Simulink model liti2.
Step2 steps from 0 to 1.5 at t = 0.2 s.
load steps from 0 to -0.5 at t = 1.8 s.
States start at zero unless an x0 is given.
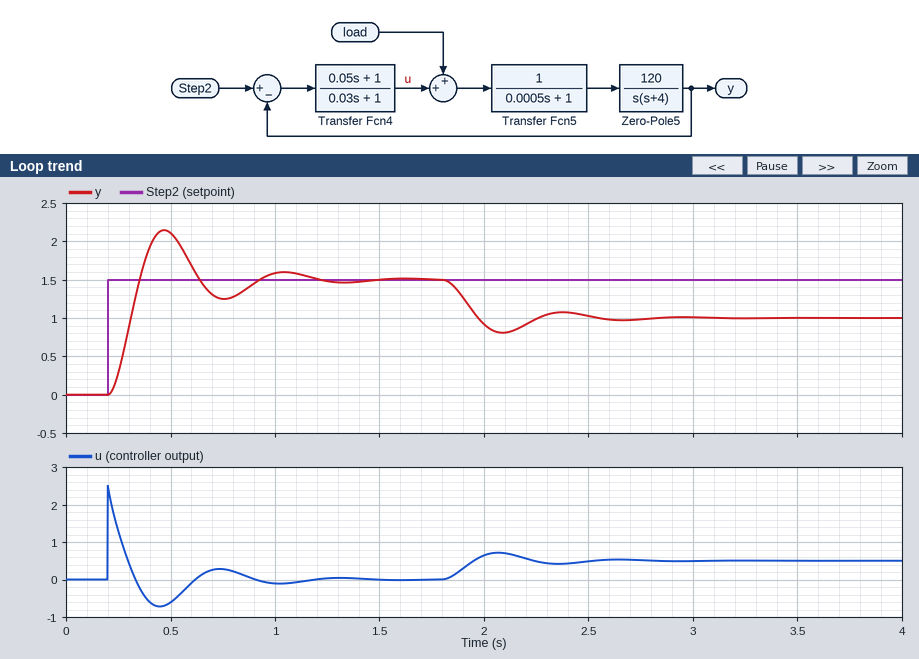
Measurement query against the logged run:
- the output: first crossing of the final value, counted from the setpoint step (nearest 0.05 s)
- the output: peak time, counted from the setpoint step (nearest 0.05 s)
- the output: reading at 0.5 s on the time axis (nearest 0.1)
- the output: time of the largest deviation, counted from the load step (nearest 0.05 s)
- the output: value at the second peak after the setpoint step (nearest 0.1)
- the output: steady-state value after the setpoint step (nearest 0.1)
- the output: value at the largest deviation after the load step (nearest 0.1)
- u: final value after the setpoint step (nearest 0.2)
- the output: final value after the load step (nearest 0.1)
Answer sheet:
0.15 s
0.25 s
2.1
0.30 s
1.6
1.5
0.8
0.0
1.0
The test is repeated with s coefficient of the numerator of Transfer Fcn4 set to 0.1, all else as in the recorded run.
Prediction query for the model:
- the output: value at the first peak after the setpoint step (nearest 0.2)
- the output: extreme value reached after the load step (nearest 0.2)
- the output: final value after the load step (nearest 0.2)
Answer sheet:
1.8
1.0
1.0
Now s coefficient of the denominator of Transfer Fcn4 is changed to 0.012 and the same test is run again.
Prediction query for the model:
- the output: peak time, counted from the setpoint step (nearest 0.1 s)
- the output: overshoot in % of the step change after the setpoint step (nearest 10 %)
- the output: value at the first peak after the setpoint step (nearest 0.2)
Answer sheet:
0.3 s
30 %
2.0
